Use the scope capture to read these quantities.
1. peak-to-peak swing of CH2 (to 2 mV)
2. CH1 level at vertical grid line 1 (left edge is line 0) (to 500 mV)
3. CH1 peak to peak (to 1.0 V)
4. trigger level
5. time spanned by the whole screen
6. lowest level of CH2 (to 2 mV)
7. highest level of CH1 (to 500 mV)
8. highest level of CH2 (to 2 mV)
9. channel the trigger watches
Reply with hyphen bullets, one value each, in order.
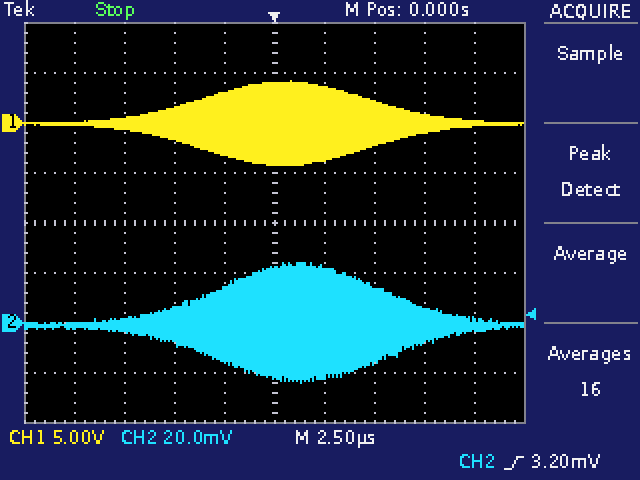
- 48 mV
- 0.0 V
- 8.0 V
- 3.20 mV
- 25 µs
- -24 mV
- 4.0 V
- 24 mV
- CH2
